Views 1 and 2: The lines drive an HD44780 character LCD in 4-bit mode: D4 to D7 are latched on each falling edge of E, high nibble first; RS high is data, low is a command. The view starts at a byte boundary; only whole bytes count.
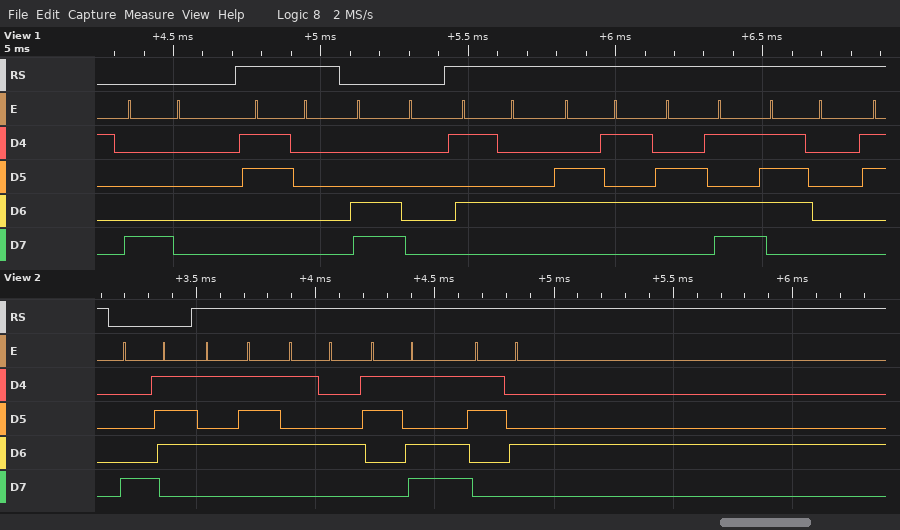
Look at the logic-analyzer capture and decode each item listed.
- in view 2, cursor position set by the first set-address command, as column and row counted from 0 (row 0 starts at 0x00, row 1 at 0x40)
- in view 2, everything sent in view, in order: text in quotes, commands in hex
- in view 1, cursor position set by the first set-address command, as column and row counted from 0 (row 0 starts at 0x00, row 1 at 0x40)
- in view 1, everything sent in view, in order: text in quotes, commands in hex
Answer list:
column 7, row 0
0x87 "WT=4"
column 0, row 0
0x80 "0" 0xC0 "Temp"
